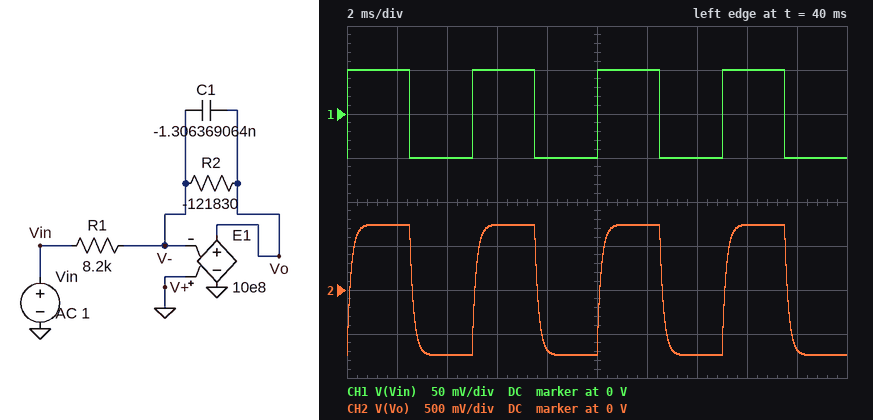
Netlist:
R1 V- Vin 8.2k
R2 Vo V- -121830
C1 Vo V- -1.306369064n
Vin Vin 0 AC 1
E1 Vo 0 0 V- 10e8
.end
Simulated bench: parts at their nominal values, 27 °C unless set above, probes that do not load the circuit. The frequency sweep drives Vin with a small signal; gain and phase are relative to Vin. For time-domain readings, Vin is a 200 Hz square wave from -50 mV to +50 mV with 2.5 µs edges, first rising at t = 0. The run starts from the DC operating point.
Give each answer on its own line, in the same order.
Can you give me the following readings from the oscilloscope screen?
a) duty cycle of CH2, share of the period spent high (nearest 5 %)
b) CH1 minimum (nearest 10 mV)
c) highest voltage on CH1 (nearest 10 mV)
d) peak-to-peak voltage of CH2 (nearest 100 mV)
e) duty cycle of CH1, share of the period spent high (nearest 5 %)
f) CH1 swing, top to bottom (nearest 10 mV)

50 %
-50 mV
50 mV
1.5 V
50 %
100 mV
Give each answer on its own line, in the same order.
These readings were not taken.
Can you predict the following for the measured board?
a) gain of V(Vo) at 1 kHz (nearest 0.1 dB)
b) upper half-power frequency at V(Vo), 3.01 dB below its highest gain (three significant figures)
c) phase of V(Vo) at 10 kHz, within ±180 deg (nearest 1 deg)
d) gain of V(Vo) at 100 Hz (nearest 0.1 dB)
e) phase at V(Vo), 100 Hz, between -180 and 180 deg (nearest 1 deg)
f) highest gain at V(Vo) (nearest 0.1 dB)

20.4 dB
1.00 kHz
-84 deg
23.4 dB
-6 deg
23.4 dB
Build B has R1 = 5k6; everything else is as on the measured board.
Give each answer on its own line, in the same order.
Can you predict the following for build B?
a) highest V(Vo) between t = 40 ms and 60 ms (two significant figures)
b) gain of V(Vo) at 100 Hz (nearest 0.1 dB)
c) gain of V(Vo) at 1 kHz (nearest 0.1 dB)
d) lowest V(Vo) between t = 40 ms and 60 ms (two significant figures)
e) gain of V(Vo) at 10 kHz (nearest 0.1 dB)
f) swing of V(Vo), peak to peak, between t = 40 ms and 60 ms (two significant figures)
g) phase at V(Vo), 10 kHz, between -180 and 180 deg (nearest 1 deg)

1.1 V
26.7 dB
23.7 dB
-1.1 V
6.7 dB
2.2 V
-84 deg
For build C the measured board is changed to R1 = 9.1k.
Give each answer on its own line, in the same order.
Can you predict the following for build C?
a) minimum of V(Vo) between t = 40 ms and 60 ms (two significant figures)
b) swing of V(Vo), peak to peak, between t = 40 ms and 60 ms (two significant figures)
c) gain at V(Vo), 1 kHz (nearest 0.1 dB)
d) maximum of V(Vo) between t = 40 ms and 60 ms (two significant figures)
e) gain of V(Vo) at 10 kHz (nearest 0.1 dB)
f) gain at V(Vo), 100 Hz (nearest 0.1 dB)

-670 mV
1.3 V
19.5 dB
670 mV
2.5 dB
22.5 dB
